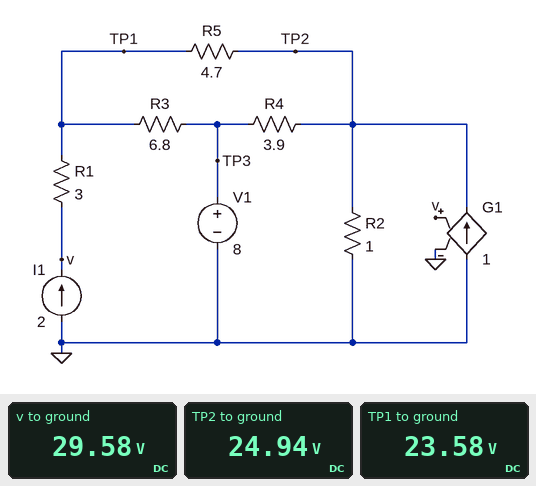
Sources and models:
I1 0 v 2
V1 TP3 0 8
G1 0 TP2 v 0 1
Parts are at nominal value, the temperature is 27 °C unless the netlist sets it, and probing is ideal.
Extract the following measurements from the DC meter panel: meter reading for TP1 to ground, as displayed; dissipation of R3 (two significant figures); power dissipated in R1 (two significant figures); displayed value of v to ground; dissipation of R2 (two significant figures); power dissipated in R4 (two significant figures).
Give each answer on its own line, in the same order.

23.58 V
36 W
12 W
29.58 V
620 W
74 W
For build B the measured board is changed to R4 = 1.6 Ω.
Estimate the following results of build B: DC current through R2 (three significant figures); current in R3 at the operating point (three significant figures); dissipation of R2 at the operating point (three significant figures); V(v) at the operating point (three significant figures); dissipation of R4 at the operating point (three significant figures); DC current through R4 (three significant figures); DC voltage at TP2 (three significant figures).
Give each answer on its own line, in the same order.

19.4 A
1.81 A
375 W
26.3 V
80.8 W
7.11 A
19.4 V
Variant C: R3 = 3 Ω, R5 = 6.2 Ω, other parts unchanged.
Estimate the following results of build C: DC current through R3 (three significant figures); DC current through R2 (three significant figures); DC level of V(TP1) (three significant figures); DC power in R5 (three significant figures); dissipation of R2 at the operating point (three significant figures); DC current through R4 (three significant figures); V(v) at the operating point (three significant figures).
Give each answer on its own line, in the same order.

2.47 A
18.3 A
15.4 V
1.35 W
335 W
2.64 A
21.4 V
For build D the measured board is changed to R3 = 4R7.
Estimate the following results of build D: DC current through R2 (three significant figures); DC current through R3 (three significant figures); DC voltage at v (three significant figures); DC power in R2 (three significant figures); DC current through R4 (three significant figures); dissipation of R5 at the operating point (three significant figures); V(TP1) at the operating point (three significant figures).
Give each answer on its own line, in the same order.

21.6 A
2.44 A
25.5 V
465 W
3.48 A
921 mW
19.5 V
